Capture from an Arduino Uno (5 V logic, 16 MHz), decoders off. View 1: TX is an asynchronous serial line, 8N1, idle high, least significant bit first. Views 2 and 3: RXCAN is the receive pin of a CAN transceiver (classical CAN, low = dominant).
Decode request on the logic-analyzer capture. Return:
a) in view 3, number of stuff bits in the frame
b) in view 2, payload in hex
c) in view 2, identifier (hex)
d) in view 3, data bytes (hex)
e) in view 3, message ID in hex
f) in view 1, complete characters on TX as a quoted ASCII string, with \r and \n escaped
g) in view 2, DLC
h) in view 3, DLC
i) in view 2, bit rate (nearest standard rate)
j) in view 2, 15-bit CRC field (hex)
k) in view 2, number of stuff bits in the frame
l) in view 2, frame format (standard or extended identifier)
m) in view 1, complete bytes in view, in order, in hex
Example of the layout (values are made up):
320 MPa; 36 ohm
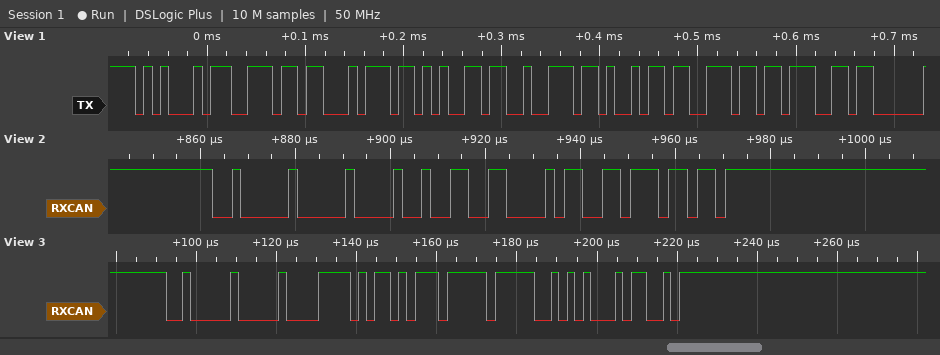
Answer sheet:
4; 4C C2; 0x200; D6 BB FF; 0x200; "Entering"; 2; 3; 500 kbit/s; 0x66ED; 2; standard; 45 6E 74 65 72 69 6E 67
